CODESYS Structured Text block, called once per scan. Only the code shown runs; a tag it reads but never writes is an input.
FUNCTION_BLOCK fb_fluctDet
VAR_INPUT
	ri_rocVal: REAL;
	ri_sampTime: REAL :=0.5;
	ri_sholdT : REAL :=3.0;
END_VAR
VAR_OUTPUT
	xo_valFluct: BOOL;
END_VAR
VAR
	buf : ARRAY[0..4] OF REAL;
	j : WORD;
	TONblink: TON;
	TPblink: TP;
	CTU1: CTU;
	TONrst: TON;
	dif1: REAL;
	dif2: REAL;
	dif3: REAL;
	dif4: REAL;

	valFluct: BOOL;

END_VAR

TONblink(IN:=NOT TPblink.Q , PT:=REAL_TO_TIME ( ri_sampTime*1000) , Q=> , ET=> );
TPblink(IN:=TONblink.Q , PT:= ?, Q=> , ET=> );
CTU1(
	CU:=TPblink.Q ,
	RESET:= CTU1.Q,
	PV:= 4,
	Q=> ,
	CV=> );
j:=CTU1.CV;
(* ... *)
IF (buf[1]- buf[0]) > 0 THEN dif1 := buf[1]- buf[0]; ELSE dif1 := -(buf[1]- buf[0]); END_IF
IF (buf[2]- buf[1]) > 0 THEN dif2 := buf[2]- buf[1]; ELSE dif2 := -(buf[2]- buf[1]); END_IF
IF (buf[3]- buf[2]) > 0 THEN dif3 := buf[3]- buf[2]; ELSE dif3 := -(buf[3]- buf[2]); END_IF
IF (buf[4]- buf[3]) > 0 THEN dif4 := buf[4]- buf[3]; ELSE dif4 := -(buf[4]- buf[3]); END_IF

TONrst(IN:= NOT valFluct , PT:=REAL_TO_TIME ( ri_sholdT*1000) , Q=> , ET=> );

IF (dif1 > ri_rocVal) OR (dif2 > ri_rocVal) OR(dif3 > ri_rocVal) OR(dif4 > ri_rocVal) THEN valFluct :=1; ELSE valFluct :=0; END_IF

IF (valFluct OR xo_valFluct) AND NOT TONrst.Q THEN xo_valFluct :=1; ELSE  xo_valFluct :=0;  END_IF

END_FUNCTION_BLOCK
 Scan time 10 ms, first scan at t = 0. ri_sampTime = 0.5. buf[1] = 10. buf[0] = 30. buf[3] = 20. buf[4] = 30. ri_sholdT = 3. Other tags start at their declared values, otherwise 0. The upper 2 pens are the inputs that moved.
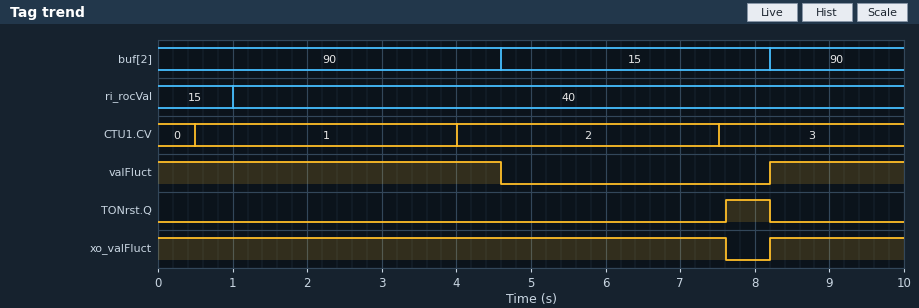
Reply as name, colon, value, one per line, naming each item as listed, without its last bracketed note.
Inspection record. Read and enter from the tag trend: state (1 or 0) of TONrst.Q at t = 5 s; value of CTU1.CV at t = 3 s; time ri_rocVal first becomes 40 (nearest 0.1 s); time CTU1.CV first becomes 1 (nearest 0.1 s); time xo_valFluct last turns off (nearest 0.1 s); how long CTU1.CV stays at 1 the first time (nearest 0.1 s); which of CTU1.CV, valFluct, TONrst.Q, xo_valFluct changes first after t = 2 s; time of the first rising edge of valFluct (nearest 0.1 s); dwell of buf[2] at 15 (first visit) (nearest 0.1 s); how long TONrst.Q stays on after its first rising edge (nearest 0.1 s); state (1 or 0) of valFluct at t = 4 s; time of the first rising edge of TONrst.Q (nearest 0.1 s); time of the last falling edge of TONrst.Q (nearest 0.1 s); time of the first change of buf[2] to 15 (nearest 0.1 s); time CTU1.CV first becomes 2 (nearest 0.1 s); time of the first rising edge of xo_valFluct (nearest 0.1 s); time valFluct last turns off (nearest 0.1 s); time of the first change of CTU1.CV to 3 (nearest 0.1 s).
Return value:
state (1 or 0) of TONrst.Q at t = 5 s: 0
value of CTU1.CV at t = 3 s: 1
time ri_rocVal first becomes 40: 1.0 s
time CTU1.CV first becomes 1: 0.5 s
time xo_valFluct last turns off: 7.6 s
how long CTU1.CV stays at 1 the first time: 3.5 s
which of CTU1.CV, valFluct, TONrst.Q, xo_valFluct changes first after t = 2 s: CTU1.CV
time of the first rising edge of valFluct: 8.2 s
dwell of buf[2] at 15 (first visit): 3.6 s
how long TONrst.Q stays on after its first rising edge: 0.6 s
state (1 or 0) of valFluct at t = 4 s: 1
time of the first rising edge of TONrst.Q: 7.6 s
time of the last falling edge of TONrst.Q: 8.2 s
time of the first change of buf[2] to 15: 4.6 s
time CTU1.CV first becomes 2: 4.0 s
time of the first rising edge of xo_valFluct: 8.2 s
time valFluct last turns off: 4.6 s
time of the first change of CTU1.CV to 3: 7.5 s
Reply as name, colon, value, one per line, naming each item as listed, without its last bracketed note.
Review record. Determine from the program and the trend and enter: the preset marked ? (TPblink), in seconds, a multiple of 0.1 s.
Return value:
the preset marked ? (TPblink), in seconds, a multiple of 0.1 s: 3.0 s
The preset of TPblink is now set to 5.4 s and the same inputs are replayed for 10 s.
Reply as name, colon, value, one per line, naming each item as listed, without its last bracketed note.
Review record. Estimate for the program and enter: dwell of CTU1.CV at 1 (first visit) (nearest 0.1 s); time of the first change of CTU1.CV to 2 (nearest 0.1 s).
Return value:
dwell of CTU1.CV at 1 (first visit): 5.9 s
time of the first change of CTU1.CV to 2: 6.4 s
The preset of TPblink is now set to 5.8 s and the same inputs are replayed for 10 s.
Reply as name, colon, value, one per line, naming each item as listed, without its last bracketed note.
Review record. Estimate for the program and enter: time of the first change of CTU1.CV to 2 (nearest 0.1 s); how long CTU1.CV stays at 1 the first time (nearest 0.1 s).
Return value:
time of the first change of CTU1.CV to 2: 6.8 s
how long CTU1.CV stays at 1 the first time: 6.3 s
